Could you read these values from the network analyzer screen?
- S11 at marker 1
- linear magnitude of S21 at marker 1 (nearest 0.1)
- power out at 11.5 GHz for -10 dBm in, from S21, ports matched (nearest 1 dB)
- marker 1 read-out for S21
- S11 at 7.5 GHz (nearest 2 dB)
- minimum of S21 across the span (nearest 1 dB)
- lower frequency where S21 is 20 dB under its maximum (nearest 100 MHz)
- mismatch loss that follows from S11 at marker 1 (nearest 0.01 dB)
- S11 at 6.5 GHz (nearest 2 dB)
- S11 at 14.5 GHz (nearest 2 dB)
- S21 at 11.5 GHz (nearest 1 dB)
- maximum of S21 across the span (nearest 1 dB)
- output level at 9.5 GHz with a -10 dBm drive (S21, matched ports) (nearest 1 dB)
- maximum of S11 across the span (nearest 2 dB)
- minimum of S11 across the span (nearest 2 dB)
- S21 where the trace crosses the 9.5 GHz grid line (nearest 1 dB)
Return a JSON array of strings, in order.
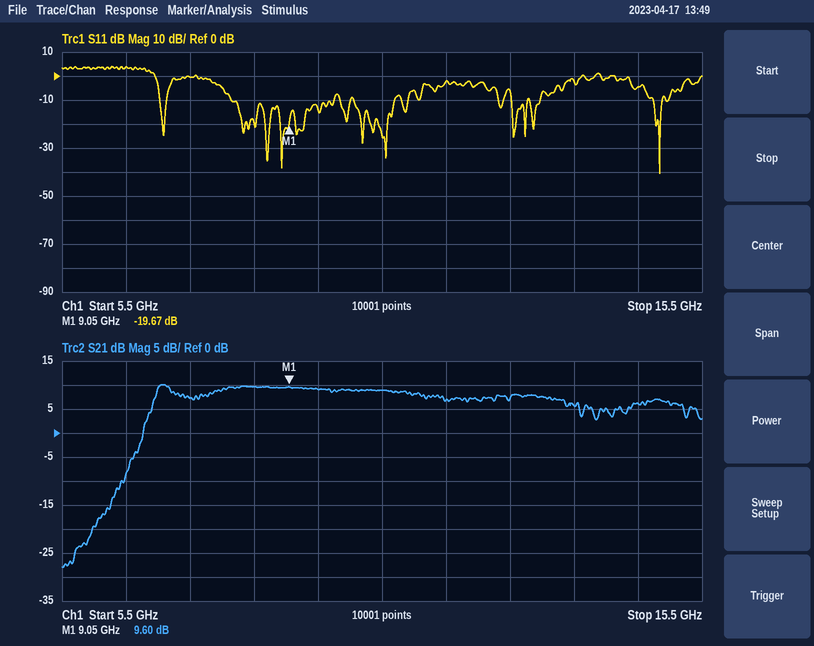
["-19.67 dB", "3.0", "-3 dBm", "9.60 dB", "0 dB", "-28 dB", "6.5 GHz", "0.05 dB", "4 dB", "-4 dB", "7 dB", "10 dB", "-1 dBm", "4 dB", "-40 dB", "9 dB"]
